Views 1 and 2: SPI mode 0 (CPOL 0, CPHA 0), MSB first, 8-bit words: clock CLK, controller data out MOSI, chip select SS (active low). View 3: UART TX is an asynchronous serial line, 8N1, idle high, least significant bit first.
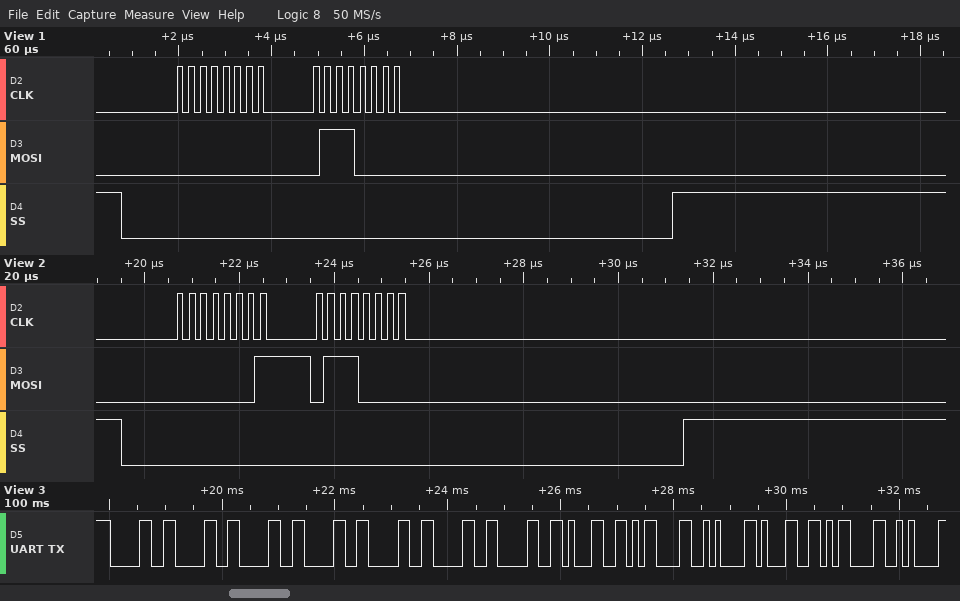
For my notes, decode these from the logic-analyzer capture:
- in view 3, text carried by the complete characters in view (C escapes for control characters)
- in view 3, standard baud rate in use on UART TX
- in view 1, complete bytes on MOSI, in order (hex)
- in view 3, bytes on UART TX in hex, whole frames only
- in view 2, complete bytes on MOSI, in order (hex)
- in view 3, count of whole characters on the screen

"00000001\r\n1\r\n"
9600 baud
00 70
30 30 30 30 30 30 30 31 0D 0A 31 0D 0A
01 70
13
